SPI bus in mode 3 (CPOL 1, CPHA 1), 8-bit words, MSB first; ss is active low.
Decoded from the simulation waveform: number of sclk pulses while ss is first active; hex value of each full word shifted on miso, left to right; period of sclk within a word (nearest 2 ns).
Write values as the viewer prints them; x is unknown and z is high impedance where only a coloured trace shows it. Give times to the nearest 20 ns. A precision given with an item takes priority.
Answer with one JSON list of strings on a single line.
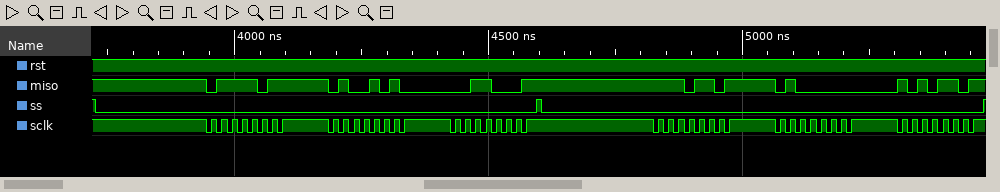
["24", "7B, 4A, 31, ED, 40, AD", "20 ns"]
